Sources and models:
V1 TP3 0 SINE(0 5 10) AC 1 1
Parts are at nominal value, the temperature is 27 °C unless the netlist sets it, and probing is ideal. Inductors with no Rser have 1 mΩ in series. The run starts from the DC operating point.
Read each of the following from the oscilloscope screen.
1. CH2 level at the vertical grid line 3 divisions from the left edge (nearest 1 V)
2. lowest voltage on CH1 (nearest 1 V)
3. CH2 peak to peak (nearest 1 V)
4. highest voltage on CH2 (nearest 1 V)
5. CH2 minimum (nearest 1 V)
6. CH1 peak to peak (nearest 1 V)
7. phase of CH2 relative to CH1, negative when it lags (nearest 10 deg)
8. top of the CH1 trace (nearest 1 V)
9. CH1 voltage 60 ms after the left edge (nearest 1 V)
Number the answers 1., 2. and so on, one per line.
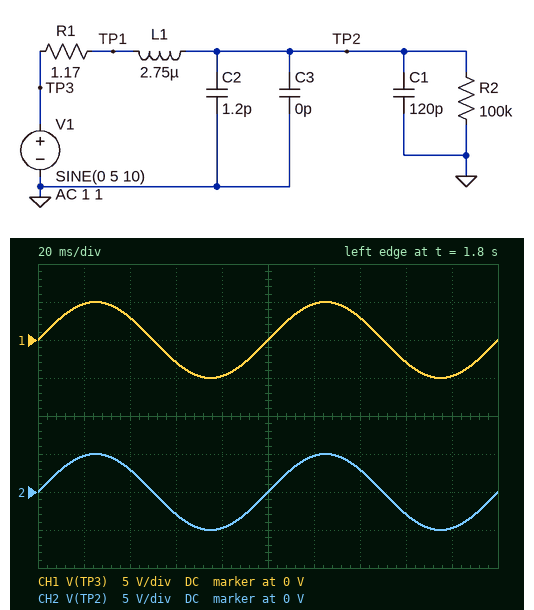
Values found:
1. -3 V
2. -5 V
3. 10 V
4. 5 V
5. -5 V
6. 10 V
7. 0 deg
8. 5 V
9. -3 V
